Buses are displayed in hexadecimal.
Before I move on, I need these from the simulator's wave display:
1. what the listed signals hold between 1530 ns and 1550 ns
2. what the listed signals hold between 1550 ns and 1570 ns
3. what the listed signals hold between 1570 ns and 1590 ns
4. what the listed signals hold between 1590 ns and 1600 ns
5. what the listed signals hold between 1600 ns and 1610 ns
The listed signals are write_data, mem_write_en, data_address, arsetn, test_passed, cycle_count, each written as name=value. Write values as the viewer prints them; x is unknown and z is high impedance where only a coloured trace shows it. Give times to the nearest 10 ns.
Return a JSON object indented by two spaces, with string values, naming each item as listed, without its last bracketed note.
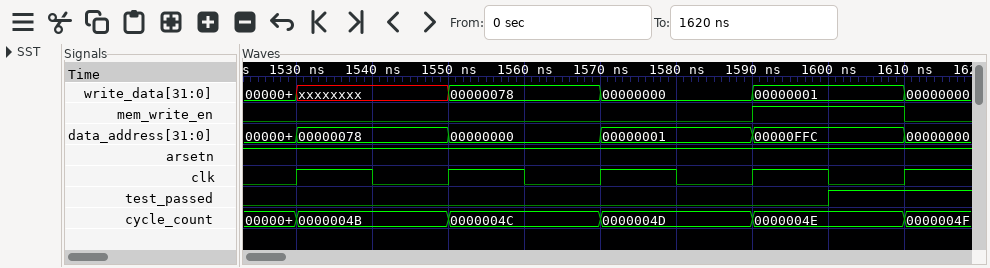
{
  "what the listed signals hold between 1530 ns and 1550 ns": "write_data=xxxxxxxx, mem_write_en=0, data_address=00000078, arsetn=1, test_passed=0, cycle_count=0000004B",
  "what the listed signals hold between 1550 ns and 1570 ns": "write_data=00000078, mem_write_en=0, data_address=00000000, arsetn=1, test_passed=0, cycle_count=0000004C",
  "what the listed signals hold between 1570 ns and 1590 ns": "write_data=00000000, mem_write_en=0, data_address=00000001, arsetn=1, test_passed=0, cycle_count=0000004D",
  "what the listed signals hold between 1590 ns and 1600 ns": "write_data=00000001, mem_write_en=1, data_address=00000FFC, arsetn=1, test_passed=0, cycle_count=0000004E",
  "what the listed signals hold between 1600 ns and 1610 ns": "write_data=00000001, mem_write_en=1, data_address=00000FFC, arsetn=1, test_passed=1, cycle_count=0000004E"
}
